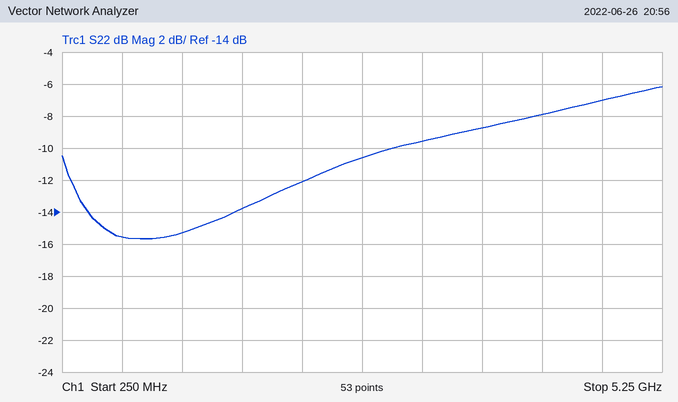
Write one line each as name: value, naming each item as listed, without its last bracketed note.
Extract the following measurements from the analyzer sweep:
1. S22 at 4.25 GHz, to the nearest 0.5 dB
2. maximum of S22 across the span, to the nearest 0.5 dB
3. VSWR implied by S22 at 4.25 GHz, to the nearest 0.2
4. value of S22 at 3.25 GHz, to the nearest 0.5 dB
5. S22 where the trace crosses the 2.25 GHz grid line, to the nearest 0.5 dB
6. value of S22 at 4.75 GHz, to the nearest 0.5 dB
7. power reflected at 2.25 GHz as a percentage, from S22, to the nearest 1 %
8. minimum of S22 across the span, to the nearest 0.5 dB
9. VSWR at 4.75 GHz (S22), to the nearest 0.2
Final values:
S22 at 4.25 GHz, to the nearest 0.5 dB: -8.0 dB
maximum of S22 across the span, to the nearest 0.5 dB: -6.0 dB
VSWR implied by S22 at 4.25 GHz, to the nearest 0.2: 2.4
value of S22 at 3.25 GHz, to the nearest 0.5 dB: -9.5 dB
S22 where the trace crosses the 2.25 GHz grid line, to the nearest 0.5 dB: -12.0 dB
value of S22 at 4.75 GHz, to the nearest 0.5 dB: -7.0 dB
power reflected at 2.25 GHz as a percentage, from S22, to the nearest 1 %: 6 %
minimum of S22 across the span, to the nearest 0.5 dB: -15.5 dB
VSWR at 4.75 GHz (S22), to the nearest 0.2: 2.6
